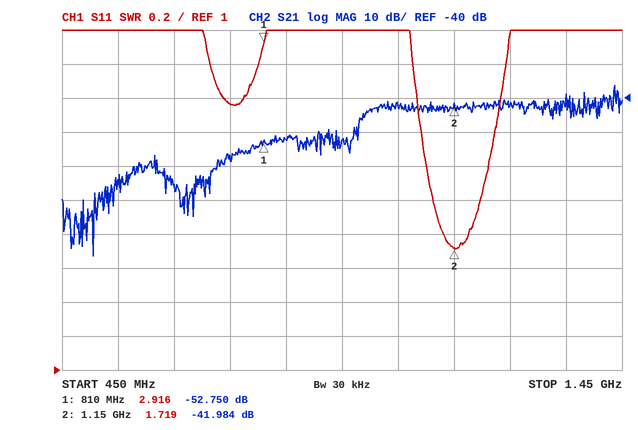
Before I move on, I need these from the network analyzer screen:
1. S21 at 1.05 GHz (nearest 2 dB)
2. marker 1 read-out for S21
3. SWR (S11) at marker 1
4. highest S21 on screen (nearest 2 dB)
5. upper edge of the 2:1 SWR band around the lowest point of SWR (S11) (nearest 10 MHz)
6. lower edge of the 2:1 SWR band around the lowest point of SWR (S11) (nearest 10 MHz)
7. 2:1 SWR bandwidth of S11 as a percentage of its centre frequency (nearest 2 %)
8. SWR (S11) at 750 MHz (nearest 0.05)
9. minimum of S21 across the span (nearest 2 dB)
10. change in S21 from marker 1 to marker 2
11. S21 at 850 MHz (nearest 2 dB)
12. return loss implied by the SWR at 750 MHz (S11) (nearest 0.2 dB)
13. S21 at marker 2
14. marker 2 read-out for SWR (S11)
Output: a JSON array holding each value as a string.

["-42 dB", "-52.750 dB", "2.916", "-36 dB", "1.20 GHz", "1.11 GHz", "8 %", "2.55", "-86 dB", "10.766 dB", "-52 dB", "7.2 dB", "-41.984 dB", "1.719"]
